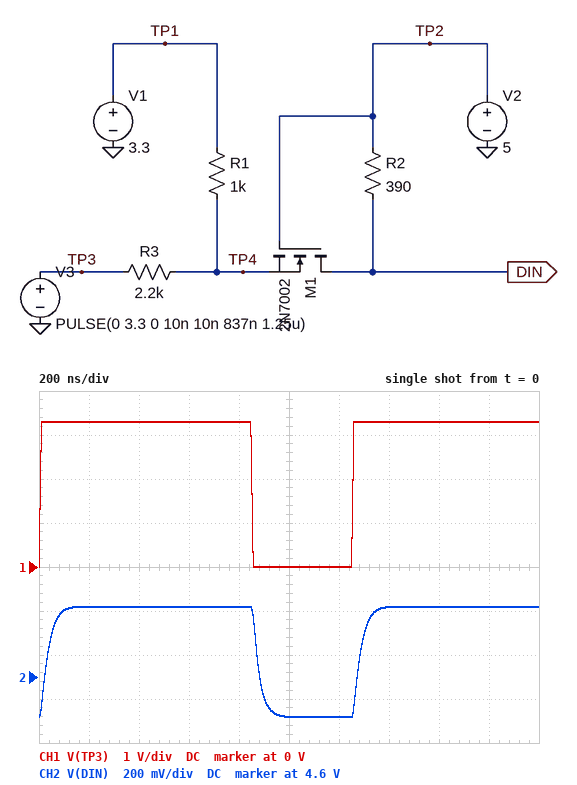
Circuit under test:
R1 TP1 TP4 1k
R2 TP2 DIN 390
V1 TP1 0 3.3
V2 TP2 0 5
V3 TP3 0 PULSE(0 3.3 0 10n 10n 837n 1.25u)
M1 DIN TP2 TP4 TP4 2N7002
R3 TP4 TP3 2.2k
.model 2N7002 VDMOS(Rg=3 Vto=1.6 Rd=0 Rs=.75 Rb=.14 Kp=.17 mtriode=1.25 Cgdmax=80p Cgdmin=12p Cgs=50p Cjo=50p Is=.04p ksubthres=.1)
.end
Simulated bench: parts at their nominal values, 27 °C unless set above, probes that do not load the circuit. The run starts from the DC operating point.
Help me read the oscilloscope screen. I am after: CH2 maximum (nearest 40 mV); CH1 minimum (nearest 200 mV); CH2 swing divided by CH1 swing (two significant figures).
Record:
4.92 V
0 V
0.15
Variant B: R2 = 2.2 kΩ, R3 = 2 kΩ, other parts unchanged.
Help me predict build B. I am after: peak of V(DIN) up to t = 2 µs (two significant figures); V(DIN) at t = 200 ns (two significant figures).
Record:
4.5 V
3.9 V
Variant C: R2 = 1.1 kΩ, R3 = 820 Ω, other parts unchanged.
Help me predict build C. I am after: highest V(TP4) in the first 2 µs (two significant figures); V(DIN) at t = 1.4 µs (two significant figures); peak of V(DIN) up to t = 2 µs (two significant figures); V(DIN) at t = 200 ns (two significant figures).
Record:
3.5 V
4.2 V
4.7 V
4.4 V
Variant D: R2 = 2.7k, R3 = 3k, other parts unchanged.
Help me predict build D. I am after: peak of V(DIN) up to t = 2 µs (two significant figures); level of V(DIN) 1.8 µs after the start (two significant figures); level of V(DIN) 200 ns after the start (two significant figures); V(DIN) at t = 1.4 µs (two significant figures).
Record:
4.4 V
4.3 V
3.8 V
3.7 V
